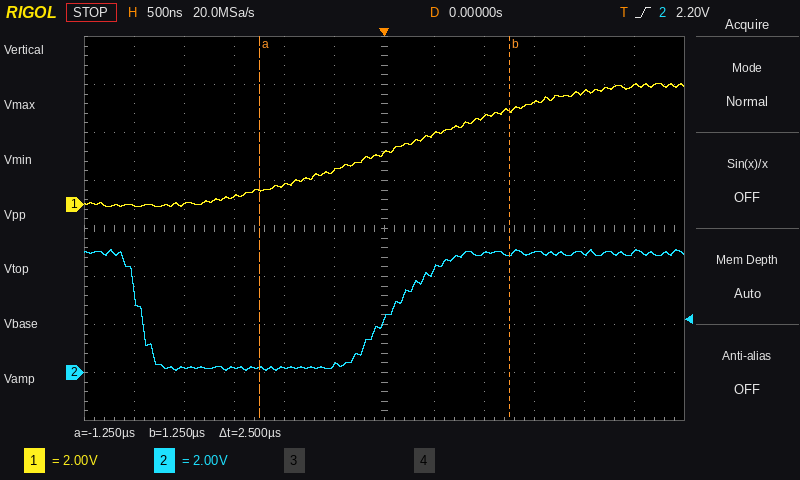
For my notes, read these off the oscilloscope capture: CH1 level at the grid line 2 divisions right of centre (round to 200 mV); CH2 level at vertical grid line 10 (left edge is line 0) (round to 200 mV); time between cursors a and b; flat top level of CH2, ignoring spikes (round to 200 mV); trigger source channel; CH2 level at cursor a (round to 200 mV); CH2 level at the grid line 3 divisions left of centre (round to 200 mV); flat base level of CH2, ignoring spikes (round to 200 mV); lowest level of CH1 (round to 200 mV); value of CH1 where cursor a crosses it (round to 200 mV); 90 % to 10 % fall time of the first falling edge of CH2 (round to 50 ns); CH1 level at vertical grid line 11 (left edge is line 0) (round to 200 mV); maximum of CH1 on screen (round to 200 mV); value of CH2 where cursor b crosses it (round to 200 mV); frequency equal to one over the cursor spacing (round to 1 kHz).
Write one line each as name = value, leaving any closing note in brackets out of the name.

CH1 level at the grid line 2 divisions right of centre = 3.6 V
CH2 level at vertical grid line 10 (left edge is line 0) = 5.0 V
time between cursors a and b = 2.5 µs
flat top level of CH2, ignoring spikes = 5.0 V
trigger source channel = CH2
CH2 level at cursor a = 200 mV
CH2 level at the grid line 3 divisions left of centre = 200 mV
flat base level of CH2, ignoring spikes = 200 mV
lowest level of CH1 = 0.0 V
value of CH1 where cursor a crosses it = 600 mV
90 % to 10 % fall time of the first falling edge of CH2 = 300 ns
CH1 level at vertical grid line 11 (left edge is line 0) = 5.0 V
maximum of CH1 on screen = 5.0 V
value of CH2 where cursor b crosses it = 5.0 V
frequency equal to one over the cursor spacing = 400 kHz
